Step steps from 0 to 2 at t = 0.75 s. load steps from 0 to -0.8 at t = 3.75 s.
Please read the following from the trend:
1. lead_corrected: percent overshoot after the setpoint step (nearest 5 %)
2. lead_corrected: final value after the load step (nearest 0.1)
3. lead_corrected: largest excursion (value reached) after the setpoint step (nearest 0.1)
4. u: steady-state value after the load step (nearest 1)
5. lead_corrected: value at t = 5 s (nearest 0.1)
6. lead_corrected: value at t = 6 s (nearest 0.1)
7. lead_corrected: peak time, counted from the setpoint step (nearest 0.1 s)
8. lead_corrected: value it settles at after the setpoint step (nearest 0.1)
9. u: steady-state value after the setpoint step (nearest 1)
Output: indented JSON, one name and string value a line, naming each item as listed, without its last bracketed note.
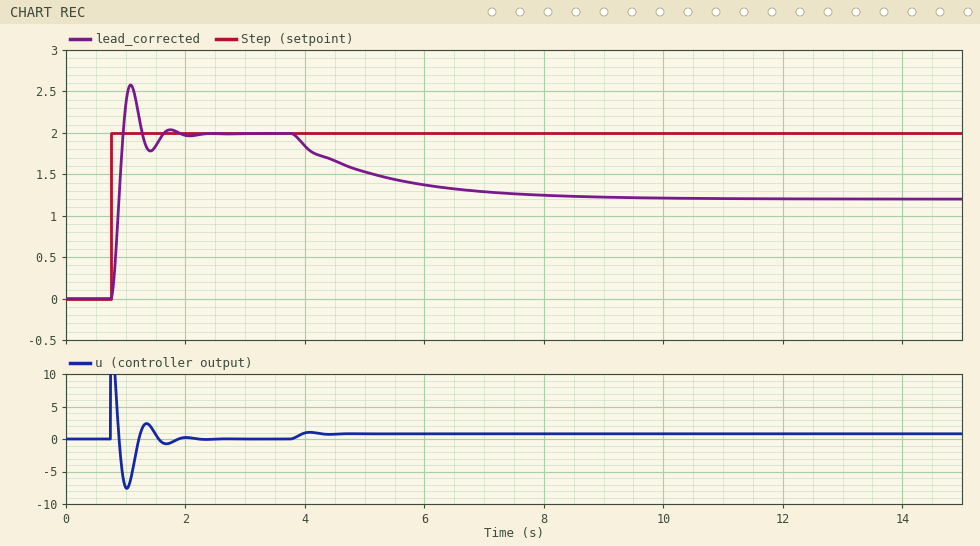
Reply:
{
  "lead_corrected: percent overshoot after the setpoint step": "30 %",
  "lead_corrected: final value after the load step": "1.2",
  "lead_corrected: largest excursion (value reached) after the setpoint step": "2.6",
  "u: steady-state value after the load step": "1",
  "lead_corrected: value at t = 5 s": "1.5",
  "lead_corrected: value at t = 6 s": "1.4",
  "lead_corrected: peak time, counted from the setpoint step": "0.3 s",
  "lead_corrected: value it settles at after the setpoint step": "2.0",
  "u: steady-state value after the setpoint step": "0"
}
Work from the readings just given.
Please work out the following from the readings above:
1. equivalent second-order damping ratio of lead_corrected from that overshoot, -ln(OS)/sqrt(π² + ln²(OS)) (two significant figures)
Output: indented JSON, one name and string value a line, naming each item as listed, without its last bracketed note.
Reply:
{
  "equivalent second-order damping ratio of lead_corrected from that overshoot, -ln(OS)/sqrt(π² + ln²(OS))": "0.36"
}
